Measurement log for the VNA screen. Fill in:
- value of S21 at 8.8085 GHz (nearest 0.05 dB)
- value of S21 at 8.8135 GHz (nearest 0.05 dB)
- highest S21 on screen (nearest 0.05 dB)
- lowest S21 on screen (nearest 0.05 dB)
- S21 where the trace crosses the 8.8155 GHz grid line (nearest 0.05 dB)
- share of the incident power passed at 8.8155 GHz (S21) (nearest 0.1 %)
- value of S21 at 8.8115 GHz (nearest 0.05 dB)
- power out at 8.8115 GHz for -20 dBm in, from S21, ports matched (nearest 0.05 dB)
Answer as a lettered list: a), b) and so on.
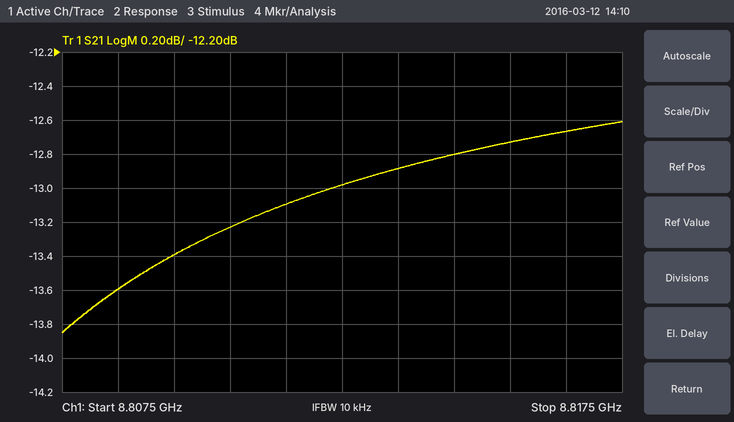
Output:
a) -13.60 dB
b) -12.90 dB
c) -12.60 dB
d) -13.85 dB
e) -12.75 dB
f) 5.3 %
g) -13.10 dB
h) -33.10 dBm
